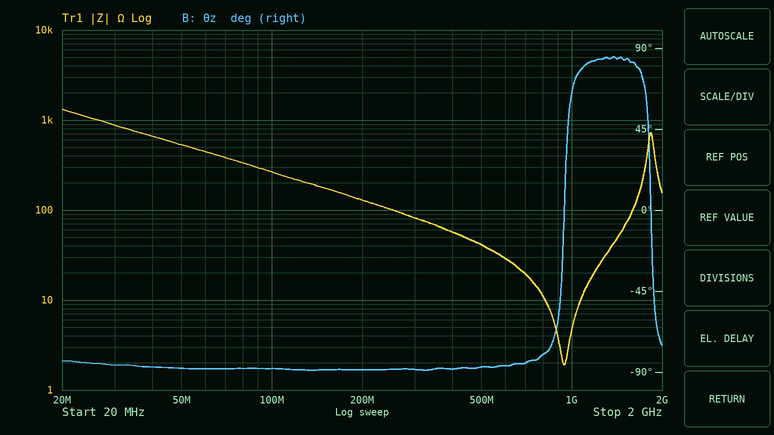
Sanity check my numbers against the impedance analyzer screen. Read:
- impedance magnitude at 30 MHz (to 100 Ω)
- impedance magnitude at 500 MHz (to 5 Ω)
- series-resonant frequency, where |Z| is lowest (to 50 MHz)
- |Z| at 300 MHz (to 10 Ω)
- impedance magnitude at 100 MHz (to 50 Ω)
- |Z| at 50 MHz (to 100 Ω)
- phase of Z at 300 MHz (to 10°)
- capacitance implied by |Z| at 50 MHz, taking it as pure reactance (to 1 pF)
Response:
900 Ω
40 Ω
950 MHz
80 Ω
250 Ω
500 Ω
-90°
6 pF
